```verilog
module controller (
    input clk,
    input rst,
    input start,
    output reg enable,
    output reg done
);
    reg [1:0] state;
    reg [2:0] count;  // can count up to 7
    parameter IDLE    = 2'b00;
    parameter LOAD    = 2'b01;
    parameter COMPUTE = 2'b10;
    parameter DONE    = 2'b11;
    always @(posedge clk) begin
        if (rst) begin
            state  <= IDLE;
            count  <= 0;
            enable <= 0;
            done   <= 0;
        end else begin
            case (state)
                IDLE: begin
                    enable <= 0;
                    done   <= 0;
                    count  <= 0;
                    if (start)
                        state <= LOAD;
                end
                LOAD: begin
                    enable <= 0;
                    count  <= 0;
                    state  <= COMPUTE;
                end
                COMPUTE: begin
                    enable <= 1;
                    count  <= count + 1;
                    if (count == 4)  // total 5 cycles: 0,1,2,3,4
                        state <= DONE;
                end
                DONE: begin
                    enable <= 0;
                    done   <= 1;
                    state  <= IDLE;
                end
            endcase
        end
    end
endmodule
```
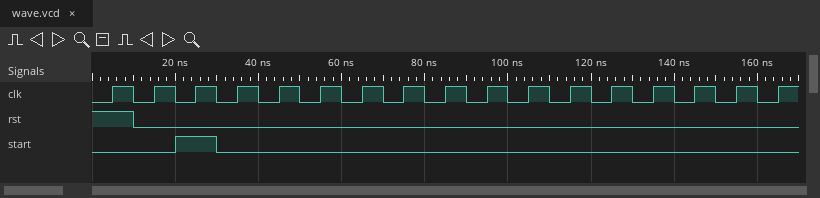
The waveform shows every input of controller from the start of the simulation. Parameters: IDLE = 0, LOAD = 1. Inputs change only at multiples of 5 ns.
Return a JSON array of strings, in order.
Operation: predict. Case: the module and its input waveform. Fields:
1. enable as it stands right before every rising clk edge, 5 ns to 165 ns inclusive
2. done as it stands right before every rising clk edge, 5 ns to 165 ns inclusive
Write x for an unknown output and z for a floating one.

["x 0 0 0 0 1 1 1 1 1 0 0 0 0 0 0 0", "x 0 0 0 0 0 0 0 0 0 1 0 0 0 0 0 0"]
